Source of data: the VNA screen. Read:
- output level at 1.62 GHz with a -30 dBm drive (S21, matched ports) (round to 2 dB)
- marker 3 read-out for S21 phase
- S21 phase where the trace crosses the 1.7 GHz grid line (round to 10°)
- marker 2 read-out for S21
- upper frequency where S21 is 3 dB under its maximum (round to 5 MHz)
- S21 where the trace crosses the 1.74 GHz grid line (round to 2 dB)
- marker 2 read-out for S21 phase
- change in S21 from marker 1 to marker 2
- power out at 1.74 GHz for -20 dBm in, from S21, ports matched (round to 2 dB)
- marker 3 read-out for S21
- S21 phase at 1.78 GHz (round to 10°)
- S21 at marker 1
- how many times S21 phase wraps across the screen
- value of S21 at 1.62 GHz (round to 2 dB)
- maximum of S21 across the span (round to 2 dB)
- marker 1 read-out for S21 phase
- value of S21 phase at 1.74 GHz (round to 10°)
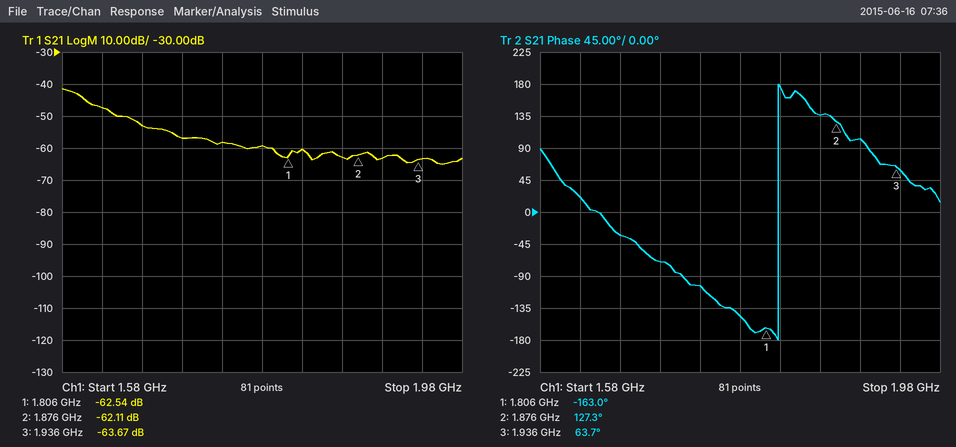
-78 dBm
63.7°
-70°
-62.11 dB
1.600 GHz
-58 dB
127.3°
0.43 dB
-78 dBm
-63.67 dB
-150°
-62.54 dB
1
-48 dB
-42 dB
-163.0°
-100°
